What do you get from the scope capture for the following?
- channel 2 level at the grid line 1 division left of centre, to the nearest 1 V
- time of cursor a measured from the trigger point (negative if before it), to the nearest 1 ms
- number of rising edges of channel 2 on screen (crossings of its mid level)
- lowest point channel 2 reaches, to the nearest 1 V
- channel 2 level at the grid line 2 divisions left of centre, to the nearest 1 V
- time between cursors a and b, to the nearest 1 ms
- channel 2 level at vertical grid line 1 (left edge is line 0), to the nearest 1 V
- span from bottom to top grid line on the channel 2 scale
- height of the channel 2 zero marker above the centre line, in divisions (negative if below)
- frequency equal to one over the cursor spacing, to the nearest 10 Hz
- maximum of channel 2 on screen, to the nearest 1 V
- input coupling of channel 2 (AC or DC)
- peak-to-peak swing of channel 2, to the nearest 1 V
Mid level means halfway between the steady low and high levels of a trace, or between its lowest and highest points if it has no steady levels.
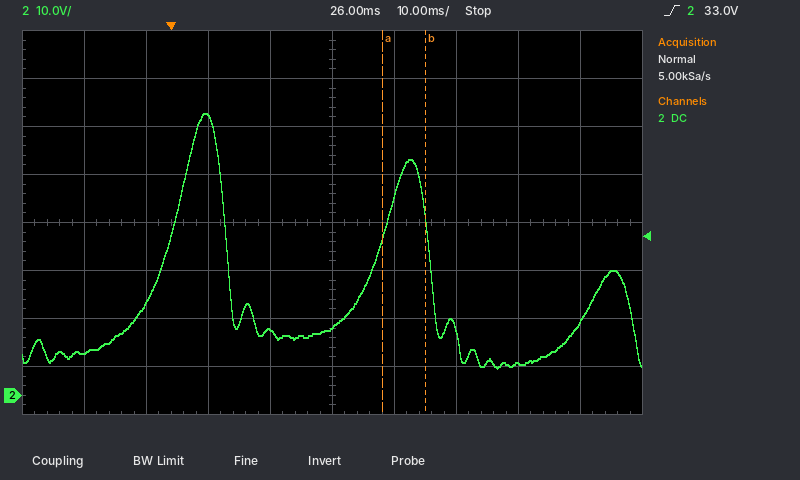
14 V
+34 ms
2
6 V
58 V
7 ms
9 V
80 V
-3.6 div
140 Hz
59 V
DC
53 V
